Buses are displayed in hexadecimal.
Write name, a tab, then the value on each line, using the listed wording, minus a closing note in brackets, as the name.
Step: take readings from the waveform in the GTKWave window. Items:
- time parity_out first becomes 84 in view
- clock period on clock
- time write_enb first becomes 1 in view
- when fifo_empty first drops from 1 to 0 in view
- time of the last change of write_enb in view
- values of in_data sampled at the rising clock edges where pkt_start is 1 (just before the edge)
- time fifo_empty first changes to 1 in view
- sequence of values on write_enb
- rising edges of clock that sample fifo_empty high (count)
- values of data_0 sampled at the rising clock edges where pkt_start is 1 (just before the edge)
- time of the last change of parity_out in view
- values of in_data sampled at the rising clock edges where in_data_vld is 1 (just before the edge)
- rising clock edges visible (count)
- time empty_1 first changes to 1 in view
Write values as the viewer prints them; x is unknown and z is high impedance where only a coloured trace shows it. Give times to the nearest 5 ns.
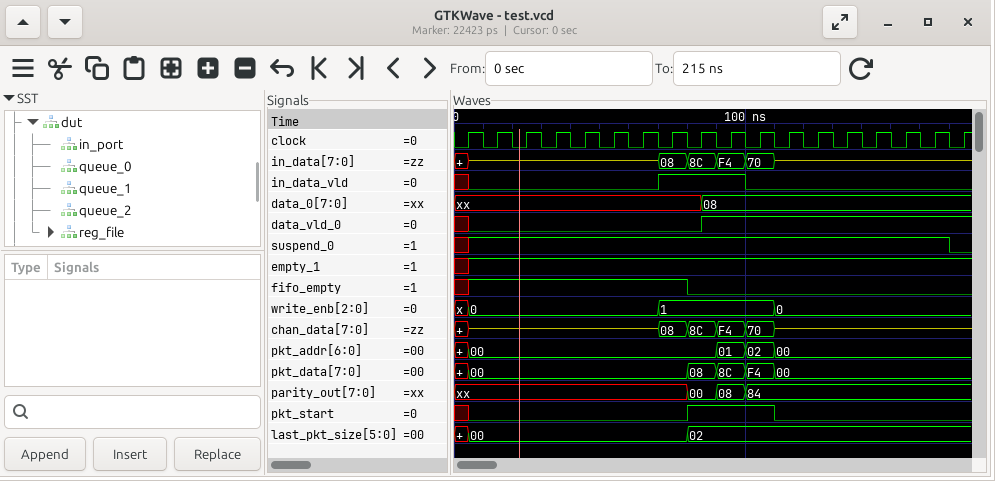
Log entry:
time parity_out first becomes 84 in view	100 ns
clock period on clock	10 ns
time write_enb first becomes 1 in view	70 ns
when fifo_empty first drops from 1 to 0 in view	80 ns
time of the last change of write_enb in view	110 ns
values of in_data sampled at the rising clock edges where pkt_start is 1	8C, F4, 70
time fifo_empty first changes to 1 in view	5 ns
sequence of values on write_enb	x, 0, 1, 0
rising edges of clock that sample fifo_empty high	7
values of data_0 sampled at the rising clock edges where pkt_start is 1	xx, 08, 08
time of the last change of parity_out in view	100 ns
values of in_data sampled at the rising clock edges where in_data_vld is 1	08, 8C, F4
rising clock edges visible	18
time empty_1 first changes to 1 in view	5 ns
